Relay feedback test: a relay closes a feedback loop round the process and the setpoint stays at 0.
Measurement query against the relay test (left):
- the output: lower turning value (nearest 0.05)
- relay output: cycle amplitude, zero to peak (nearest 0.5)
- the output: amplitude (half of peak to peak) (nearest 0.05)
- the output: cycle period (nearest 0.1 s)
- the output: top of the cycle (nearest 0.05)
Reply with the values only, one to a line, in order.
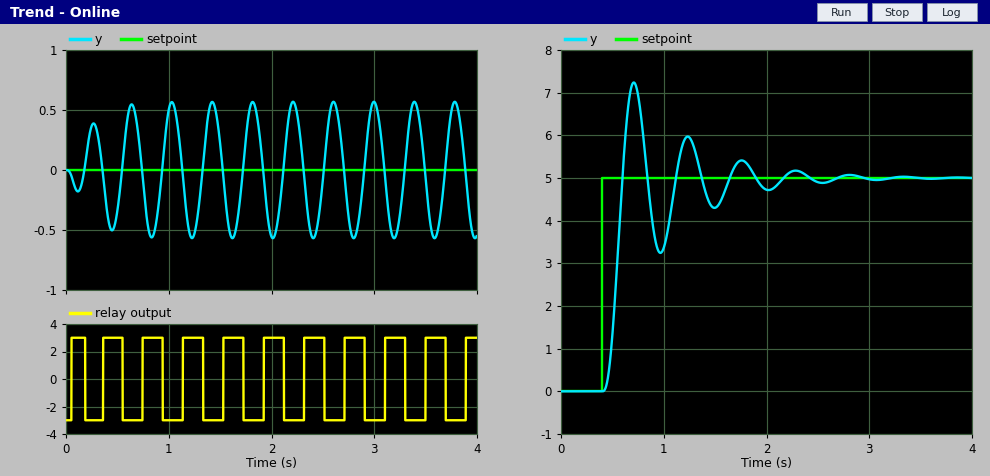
-0.55
3.0
0.55
0.4 s
0.55
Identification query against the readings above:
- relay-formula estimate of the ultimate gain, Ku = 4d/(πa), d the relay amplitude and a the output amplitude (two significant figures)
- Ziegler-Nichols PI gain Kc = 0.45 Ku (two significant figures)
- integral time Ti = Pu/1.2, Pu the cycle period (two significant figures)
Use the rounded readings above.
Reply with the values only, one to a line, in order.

6.9
3.1
0.33 s
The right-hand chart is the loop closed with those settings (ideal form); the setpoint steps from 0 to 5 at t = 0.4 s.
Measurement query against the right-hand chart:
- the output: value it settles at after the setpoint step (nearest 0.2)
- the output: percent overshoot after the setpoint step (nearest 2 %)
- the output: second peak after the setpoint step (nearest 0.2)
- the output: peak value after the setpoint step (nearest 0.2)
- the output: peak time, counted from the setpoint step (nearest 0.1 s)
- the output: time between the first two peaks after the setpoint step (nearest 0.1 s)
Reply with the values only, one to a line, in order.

5.0
44 %
6.0
7.2
0.3 s
0.5 s
